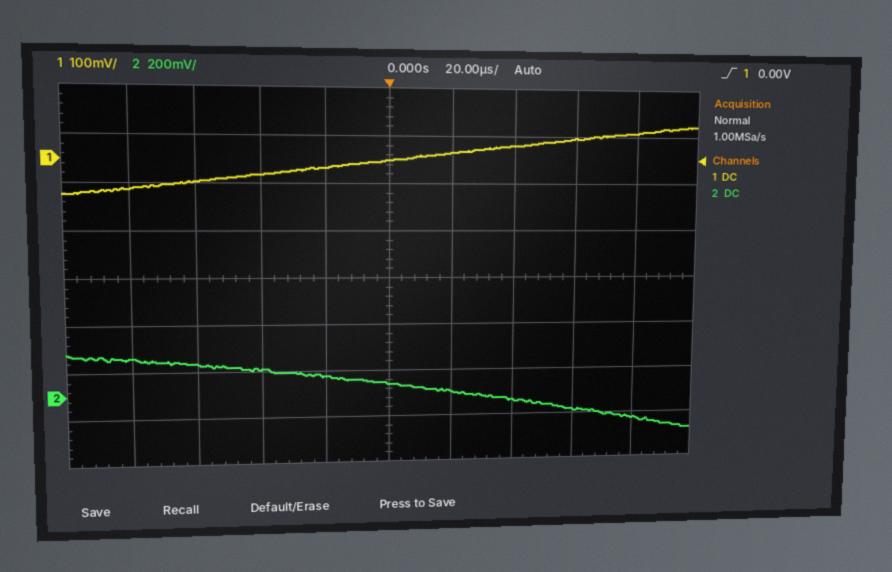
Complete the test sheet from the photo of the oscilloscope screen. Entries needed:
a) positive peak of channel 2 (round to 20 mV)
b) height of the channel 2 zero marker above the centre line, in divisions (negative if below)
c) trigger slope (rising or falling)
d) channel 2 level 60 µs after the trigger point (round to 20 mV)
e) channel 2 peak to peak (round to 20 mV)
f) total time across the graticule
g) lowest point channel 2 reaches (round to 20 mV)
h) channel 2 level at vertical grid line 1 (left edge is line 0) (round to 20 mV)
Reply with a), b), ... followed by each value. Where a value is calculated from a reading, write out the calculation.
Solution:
a) 180 mV
b) -2.5 div
c) rising
d) -80 mV
e) 180 mV − (-180 mV) = 360 mV
f) 200 µs
g) -180 mV
h) 160 mV
